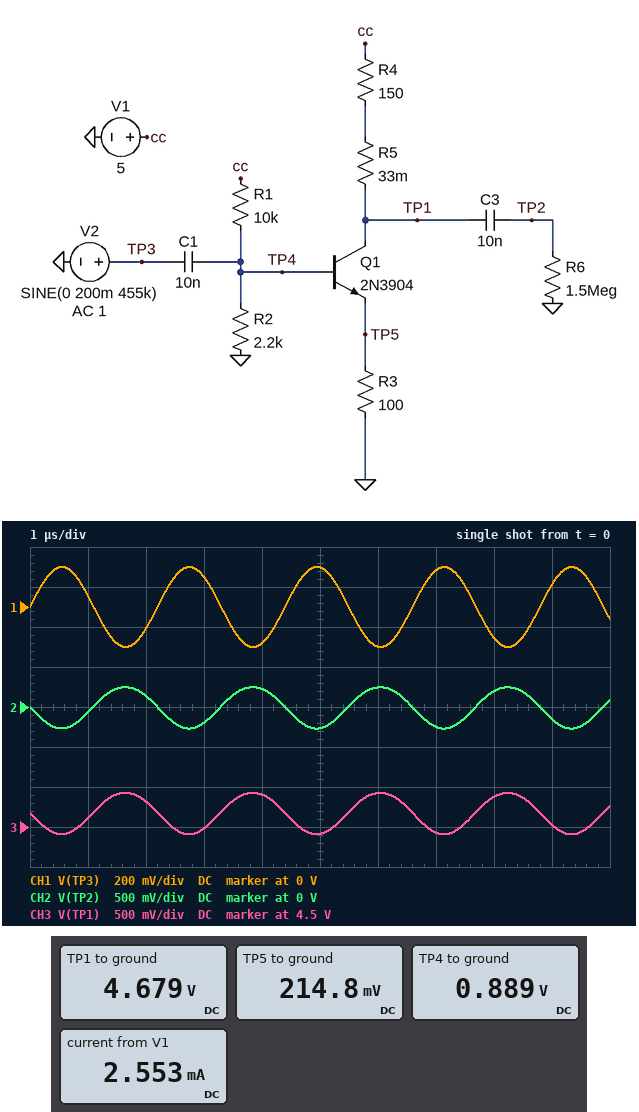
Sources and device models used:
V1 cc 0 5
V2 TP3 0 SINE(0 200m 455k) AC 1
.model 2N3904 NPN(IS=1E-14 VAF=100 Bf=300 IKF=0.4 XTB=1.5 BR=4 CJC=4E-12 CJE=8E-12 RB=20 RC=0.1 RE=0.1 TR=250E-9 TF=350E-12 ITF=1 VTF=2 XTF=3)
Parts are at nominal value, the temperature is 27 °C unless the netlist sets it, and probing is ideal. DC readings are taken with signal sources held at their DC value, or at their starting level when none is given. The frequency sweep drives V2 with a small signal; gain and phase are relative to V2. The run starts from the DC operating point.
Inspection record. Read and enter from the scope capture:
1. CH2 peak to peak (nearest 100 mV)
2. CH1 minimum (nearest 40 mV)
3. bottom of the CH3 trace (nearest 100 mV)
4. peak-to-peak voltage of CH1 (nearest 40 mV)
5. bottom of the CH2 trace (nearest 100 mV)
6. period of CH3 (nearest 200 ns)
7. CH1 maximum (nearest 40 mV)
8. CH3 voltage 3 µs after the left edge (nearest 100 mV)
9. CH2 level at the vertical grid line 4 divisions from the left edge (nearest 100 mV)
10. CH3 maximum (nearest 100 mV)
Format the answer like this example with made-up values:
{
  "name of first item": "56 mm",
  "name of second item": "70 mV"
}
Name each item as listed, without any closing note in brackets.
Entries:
{
  "CH2 peak to peak": "500 mV",
  "CH1 minimum": "-200 mV",
  "bottom of the CH3 trace": "4.4 V",
  "peak-to-peak voltage of CH1": "400 mV",
  "bottom of the CH2 trace": "-300 mV",
  "period of CH3": "2.2 µs",
  "CH1 maximum": "200 mV",
  "CH3 voltage 3 µs after the left edge": "4.5 V",
  "CH2 level at the vertical grid line 4 divisions from the left edge": "200 mV",
  "CH3 maximum": "4.9 V"
}
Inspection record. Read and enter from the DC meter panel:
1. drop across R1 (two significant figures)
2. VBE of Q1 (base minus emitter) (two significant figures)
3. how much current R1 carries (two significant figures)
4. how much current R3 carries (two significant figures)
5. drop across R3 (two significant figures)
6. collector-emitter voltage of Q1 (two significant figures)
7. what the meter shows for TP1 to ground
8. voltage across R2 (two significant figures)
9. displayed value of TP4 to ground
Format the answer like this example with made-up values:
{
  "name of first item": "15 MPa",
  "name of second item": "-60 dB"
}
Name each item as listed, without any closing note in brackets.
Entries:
{
  "drop across R1": "4.1 V",
  "VBE of Q1 (base minus emitter)": "670 mV",
  "how much current R1 carries": "410 µA",
  "how much current R3 carries": "2.1 mA",
  "drop across R3": "210 mV",
  "collector-emitter voltage of Q1": "4.5 V",
  "what the meter shows for TP1 to ground": "4.679 V",
  "voltage across R2": "890 mV",
  "displayed value of TP4 to ground": "0.889 V"
}
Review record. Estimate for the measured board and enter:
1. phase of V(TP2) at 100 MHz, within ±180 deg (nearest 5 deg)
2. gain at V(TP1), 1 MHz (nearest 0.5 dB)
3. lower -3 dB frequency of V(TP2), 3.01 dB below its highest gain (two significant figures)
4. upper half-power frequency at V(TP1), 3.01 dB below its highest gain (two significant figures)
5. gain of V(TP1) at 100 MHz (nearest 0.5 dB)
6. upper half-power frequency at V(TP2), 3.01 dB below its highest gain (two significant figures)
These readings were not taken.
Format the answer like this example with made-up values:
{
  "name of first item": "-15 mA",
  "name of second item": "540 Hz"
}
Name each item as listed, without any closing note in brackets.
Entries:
{
  "phase of V(TP2) at 100 MHz, within ±180 deg": "140 deg",
  "gain at V(TP1), 1 MHz": "2.5 dB",
  "lower -3 dB frequency of V(TP2), 3.01 dB below its highest gain": "9.3 kHz",
  "upper half-power frequency at V(TP1), 3.01 dB below its highest gain": "480 MHz",
  "gain of V(TP1) at 100 MHz": "2.0 dB",
  "upper half-power frequency at V(TP2), 3.01 dB below its highest gain": "480 MHz"
}
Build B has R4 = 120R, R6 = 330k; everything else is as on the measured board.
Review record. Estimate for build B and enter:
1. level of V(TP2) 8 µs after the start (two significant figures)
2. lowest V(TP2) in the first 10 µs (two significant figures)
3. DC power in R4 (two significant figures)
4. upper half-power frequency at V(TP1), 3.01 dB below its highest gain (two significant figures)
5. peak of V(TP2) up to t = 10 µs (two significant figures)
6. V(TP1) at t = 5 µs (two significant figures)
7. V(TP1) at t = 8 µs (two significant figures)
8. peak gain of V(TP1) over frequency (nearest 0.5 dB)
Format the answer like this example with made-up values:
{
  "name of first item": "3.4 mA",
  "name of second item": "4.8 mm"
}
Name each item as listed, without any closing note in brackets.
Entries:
{
  "level of V(TP2) 8 µs after the start": "160 mV",
  "lowest V(TP2) in the first 10 µs": "-220 mV",
  "DC power in R4": "550 µW",
  "upper half-power frequency at V(TP1), 3.01 dB below its highest gain": "1.4 GHz",
  "peak of V(TP2) up to t = 10 µs": "200 mV",
  "V(TP1) at t = 5 µs": "4.5 V",
  "V(TP1) at t = 8 µs": "4.9 V",
  "peak gain of V(TP1) over frequency": "0.5 dB"
}
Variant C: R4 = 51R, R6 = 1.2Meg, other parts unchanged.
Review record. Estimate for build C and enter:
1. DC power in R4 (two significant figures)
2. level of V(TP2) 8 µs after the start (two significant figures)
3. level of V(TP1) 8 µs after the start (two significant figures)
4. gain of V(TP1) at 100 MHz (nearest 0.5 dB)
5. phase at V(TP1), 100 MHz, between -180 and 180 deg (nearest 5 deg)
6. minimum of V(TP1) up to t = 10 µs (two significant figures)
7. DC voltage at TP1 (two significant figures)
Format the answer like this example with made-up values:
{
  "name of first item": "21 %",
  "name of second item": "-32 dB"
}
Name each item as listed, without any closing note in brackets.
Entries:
{
  "DC power in R4": "230 µW",
  "level of V(TP2) 8 µs after the start": "68 mV",
  "level of V(TP1) 8 µs after the start": "5.0 V",
  "gain of V(TP1) at 100 MHz": "-7.0 dB",
  "phase at V(TP1), 100 MHz, between -180 and 180 deg": "145 deg",
  "minimum of V(TP1) up to t = 10 µs": "4.8 V",
  "DC voltage at TP1": "4.9 V"
}
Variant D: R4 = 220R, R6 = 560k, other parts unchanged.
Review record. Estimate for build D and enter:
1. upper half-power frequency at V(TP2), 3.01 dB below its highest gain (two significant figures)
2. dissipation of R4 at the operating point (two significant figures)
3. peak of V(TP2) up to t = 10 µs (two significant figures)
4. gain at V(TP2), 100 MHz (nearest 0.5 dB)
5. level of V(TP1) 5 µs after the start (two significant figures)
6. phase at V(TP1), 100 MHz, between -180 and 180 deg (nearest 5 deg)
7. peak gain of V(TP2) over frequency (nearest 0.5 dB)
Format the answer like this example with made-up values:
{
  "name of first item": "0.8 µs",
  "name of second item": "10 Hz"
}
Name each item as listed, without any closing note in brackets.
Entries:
{
  "upper half-power frequency at V(TP2), 3.01 dB below its highest gain": "270 MHz",
  "dissipation of R4 at the operating point": "1.0 mW",
  "peak of V(TP2) up to t = 10 µs": "360 mV",
  "gain at V(TP2), 100 MHz": "5.0 dB",
  "level of V(TP1) 5 µs after the start": "4.1 V",
  "phase at V(TP1), 100 MHz, between -180 and 180 deg": "130 deg",
  "peak gain of V(TP2) over frequency": "6.0 dB"
}
